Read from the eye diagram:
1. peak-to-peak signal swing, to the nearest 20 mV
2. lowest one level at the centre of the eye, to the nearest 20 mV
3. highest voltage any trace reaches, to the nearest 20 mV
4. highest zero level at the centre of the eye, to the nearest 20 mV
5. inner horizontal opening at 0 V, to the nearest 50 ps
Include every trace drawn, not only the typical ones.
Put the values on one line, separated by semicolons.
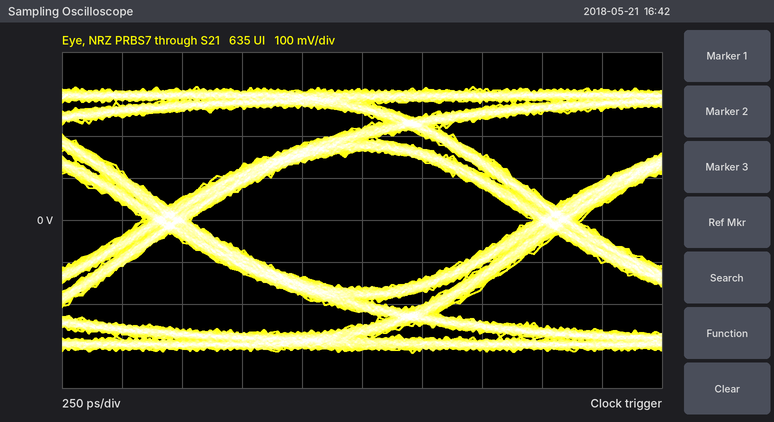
640 mV; 160 mV; 320 mV; -160 mV; 1.45 ns
